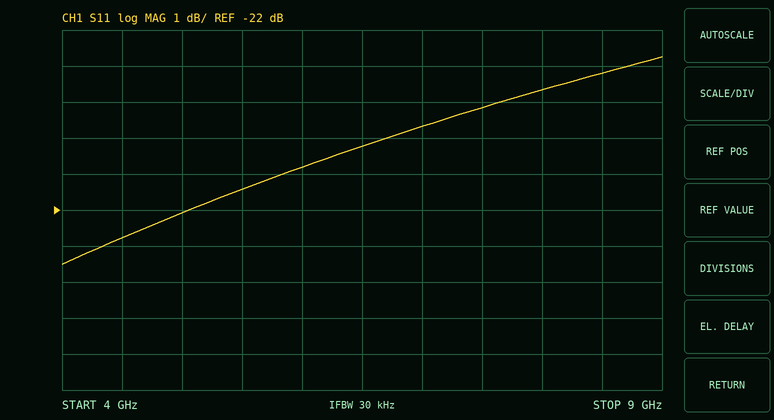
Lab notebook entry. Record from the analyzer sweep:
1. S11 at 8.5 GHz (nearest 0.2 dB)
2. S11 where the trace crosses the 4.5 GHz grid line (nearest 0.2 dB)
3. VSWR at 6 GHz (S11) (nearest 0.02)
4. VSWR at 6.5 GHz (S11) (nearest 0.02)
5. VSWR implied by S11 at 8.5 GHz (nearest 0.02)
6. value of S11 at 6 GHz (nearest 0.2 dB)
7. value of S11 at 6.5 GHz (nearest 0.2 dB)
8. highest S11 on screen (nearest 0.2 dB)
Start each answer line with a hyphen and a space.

- -18.2 dB
- -22.8 dB
- 1.20
- 1.22
- 1.28
- -20.8 dB
- -20.2 dB
- -17.8 dB
